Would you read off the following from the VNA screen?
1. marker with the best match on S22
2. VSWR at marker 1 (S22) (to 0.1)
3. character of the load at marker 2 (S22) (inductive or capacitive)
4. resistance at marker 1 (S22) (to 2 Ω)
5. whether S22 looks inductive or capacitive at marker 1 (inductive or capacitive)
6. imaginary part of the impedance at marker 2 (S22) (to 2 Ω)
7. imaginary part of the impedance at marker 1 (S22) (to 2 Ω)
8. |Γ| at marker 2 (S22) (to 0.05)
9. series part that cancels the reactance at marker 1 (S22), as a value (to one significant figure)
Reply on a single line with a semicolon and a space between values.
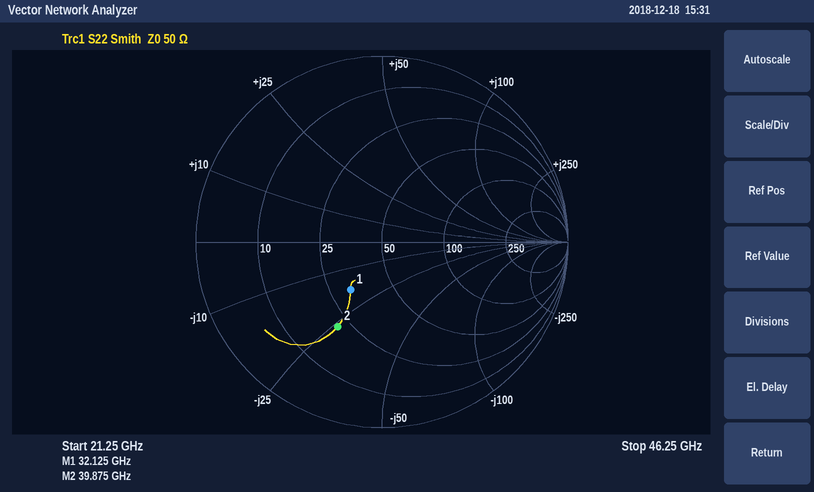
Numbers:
marker 1; 1.9; capacitive; 32 Ω; capacitive; -26 Ω; -18 Ω; 0.50; 90 pH
